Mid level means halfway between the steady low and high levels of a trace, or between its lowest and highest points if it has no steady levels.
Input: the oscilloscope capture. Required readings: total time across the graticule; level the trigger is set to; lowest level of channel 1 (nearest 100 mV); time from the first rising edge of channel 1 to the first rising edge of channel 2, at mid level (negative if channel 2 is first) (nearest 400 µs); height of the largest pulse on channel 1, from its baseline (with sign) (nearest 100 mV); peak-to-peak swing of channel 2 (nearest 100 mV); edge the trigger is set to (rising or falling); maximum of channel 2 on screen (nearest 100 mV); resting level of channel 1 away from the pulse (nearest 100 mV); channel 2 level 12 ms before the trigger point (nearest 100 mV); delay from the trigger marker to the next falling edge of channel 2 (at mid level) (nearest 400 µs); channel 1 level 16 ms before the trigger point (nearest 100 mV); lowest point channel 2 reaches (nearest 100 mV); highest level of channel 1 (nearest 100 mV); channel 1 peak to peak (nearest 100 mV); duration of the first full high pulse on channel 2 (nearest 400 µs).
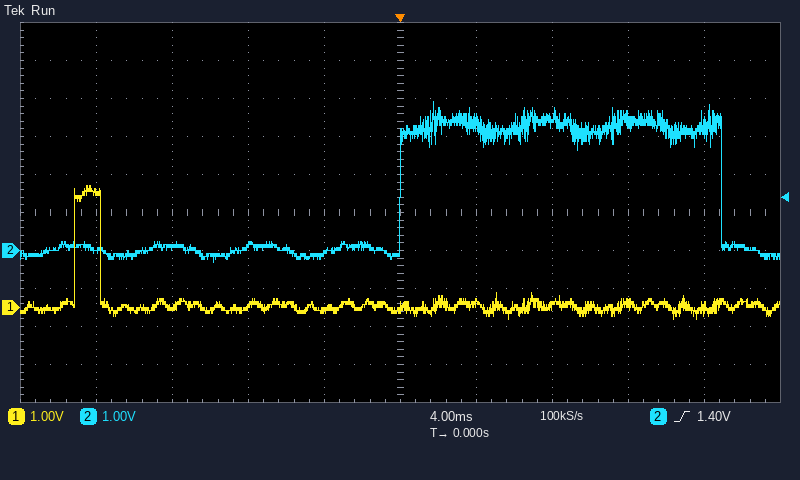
40 ms
1.40 V
-300 mV
+17.2 ms
+3.2 V
4.2 V
rising
3.9 V
0.0 V
100 mV
16.8 ms
3.0 V
-300 mV
3.2 V
3.5 V
16.8 ms
